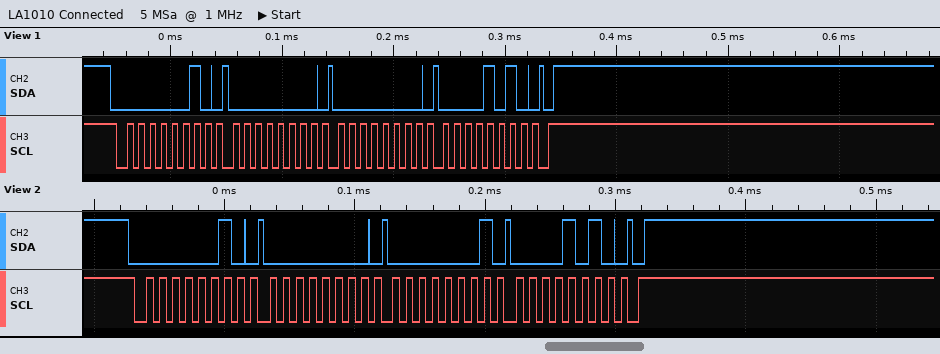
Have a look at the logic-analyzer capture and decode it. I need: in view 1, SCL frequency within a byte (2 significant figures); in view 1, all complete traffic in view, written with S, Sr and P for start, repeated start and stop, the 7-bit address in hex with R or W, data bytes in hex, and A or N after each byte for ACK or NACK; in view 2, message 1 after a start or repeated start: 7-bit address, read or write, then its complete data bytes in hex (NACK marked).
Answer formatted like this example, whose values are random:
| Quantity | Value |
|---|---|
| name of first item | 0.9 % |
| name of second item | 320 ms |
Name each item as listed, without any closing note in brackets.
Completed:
| Quantity | Value |
|---|---|
| in view 1, SCL frequency within a byte | 100 kHz |
| in view 1, all complete traffic in view, written with S, Sr and P for start, repeated start and stop, the 7-bit address in hex with R or W, data bytes in hex, and A or N after each byte for ACK or NACK | S 01W A 00 A 00 A 0A A P |
| in view 2, message 1 after a start or repeated start: 7-bit address, read or write, then its complete data bytes in hex | 0x01 write: 00 01 0A |
